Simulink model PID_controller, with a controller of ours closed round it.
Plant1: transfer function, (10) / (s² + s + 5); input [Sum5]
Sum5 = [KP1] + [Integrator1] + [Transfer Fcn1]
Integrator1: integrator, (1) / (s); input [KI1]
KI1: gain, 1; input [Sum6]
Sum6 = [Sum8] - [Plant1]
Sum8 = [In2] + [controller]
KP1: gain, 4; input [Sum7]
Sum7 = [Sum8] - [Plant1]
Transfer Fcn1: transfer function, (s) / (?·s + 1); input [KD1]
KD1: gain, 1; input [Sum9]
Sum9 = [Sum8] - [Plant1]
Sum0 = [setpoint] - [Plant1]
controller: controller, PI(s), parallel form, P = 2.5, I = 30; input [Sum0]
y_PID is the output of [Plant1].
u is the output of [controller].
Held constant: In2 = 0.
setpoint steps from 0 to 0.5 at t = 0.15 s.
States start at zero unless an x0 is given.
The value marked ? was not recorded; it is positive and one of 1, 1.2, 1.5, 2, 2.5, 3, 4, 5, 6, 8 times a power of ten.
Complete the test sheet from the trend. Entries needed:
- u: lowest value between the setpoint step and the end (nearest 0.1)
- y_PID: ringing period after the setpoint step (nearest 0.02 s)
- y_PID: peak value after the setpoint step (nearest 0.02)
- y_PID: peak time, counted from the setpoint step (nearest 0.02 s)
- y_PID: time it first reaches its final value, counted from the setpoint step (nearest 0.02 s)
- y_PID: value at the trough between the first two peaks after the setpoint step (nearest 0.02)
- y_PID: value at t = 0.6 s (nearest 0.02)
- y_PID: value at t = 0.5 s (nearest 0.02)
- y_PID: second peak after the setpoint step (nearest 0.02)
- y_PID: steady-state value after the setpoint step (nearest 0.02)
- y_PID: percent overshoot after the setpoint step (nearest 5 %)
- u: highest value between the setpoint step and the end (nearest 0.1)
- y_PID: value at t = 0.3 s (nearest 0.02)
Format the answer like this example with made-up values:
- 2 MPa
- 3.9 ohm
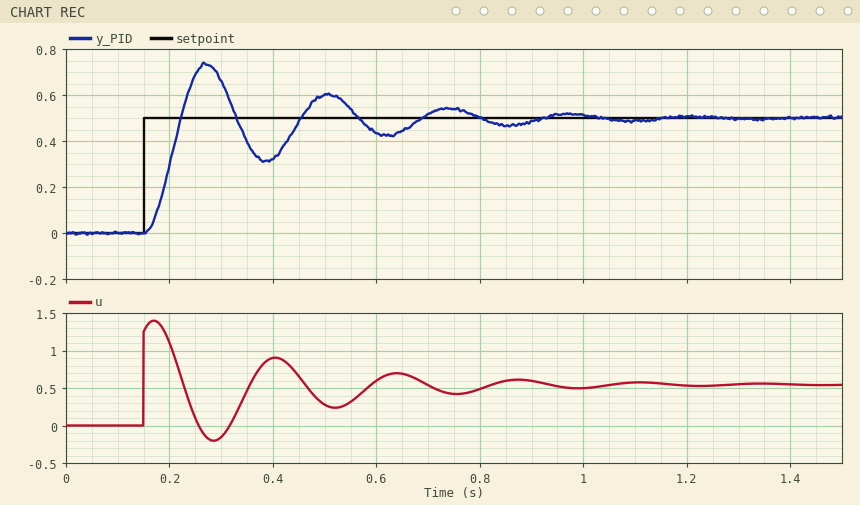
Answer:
- -0.2
- 0.24 s
- 0.74
- 0.12 s
- 0.08 s
- 0.32
- 0.44
- 0.60
- 0.60
- 0.50
- 45 %
- 1.4
- 0.66
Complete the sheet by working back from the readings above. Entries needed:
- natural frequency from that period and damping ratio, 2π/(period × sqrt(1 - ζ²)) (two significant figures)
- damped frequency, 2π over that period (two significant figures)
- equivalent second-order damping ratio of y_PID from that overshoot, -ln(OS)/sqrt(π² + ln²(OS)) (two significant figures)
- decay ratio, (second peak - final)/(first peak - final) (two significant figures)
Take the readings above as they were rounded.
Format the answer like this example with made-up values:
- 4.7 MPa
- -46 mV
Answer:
- 27 rad/s
- 26 rad/s
- 0.25
- 0.42
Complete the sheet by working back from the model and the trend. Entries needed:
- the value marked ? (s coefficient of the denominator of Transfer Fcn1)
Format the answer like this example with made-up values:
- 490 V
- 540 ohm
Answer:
- 0.05
